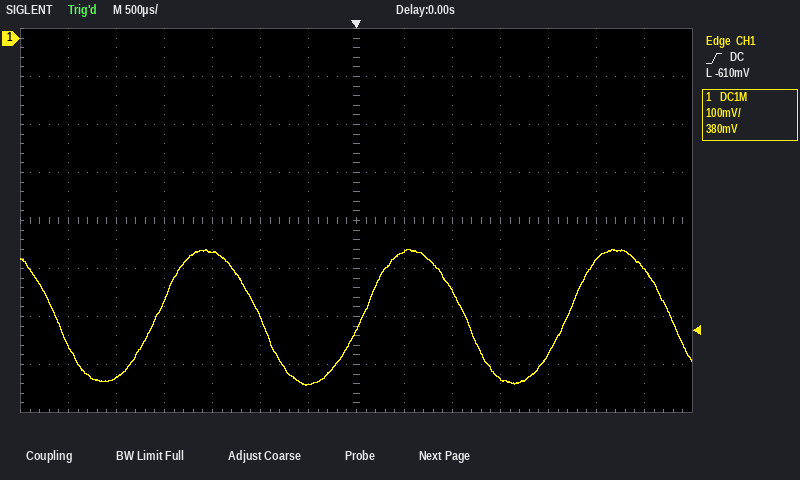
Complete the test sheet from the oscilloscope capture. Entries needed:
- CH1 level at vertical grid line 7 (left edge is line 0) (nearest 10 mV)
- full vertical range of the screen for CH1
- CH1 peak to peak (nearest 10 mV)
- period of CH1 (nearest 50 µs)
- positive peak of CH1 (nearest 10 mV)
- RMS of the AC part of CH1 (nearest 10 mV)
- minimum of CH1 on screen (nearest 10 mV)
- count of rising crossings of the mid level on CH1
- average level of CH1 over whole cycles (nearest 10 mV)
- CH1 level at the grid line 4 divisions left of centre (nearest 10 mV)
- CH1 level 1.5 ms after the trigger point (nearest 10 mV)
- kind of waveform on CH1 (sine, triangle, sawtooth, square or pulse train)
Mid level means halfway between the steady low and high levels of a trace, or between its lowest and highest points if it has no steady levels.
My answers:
-610 mV
800 mV
280 mV
2.15 ms
-440 mV
100 mV
-720 mV
3
-580 mV
-550 mV
-710 mV
sine
